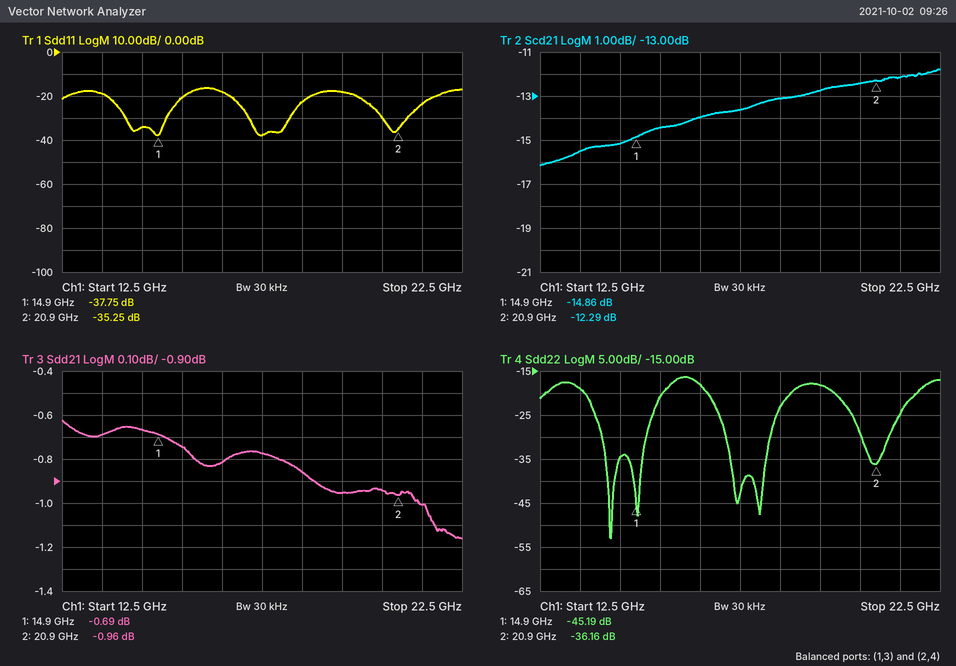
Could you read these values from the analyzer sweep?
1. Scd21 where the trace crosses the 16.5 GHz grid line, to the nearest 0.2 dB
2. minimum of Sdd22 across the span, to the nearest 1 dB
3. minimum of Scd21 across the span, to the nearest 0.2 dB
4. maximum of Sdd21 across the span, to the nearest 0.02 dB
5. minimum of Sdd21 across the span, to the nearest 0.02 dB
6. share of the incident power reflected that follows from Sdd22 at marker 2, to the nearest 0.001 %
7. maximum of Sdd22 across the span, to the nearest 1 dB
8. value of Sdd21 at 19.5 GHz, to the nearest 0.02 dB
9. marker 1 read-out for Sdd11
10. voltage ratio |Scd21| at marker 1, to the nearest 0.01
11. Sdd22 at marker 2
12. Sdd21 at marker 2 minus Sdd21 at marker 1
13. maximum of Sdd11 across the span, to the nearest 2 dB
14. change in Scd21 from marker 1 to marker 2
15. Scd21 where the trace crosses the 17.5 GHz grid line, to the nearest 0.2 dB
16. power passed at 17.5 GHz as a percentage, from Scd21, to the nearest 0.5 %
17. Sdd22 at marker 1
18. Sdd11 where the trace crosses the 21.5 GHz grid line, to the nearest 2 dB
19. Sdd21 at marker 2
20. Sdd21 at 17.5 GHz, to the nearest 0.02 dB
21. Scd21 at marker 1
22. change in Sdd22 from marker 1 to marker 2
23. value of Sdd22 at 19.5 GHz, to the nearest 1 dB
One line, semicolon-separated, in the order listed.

-14.0 dB; -53 dB; -16.2 dB; -0.62 dB; -1.16 dB; 0.024 %; -16 dB; -0.96 dB; -37.75 dB; 0.18; -36.16 dB; -0.27 dB; -16 dB; 2.57 dB; -13.6 dB; 4.5 %; -45.19 dB; -24 dB; -0.96 dB; -0.78 dB; -14.86 dB; 9.03 dB; -18 dB
